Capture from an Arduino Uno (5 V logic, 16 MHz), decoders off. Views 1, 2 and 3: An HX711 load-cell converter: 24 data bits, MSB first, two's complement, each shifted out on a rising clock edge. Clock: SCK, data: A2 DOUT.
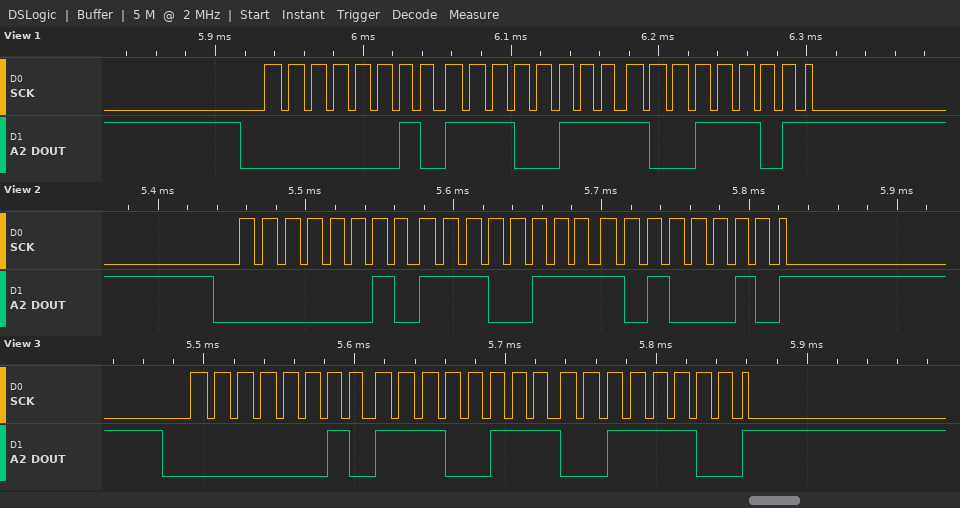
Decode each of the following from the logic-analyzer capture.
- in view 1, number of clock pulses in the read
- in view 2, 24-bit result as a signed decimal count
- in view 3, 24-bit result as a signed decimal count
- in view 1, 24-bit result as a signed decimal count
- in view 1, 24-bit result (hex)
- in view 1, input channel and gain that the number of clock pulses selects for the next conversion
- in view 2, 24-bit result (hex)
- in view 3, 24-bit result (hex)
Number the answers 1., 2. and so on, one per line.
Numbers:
1. 25
2. 190370
3. 190268
4. 190365
5. 0x02E79D
6. channel A, gain 128
7. 0x02E7A2
8. 0x02E73C
